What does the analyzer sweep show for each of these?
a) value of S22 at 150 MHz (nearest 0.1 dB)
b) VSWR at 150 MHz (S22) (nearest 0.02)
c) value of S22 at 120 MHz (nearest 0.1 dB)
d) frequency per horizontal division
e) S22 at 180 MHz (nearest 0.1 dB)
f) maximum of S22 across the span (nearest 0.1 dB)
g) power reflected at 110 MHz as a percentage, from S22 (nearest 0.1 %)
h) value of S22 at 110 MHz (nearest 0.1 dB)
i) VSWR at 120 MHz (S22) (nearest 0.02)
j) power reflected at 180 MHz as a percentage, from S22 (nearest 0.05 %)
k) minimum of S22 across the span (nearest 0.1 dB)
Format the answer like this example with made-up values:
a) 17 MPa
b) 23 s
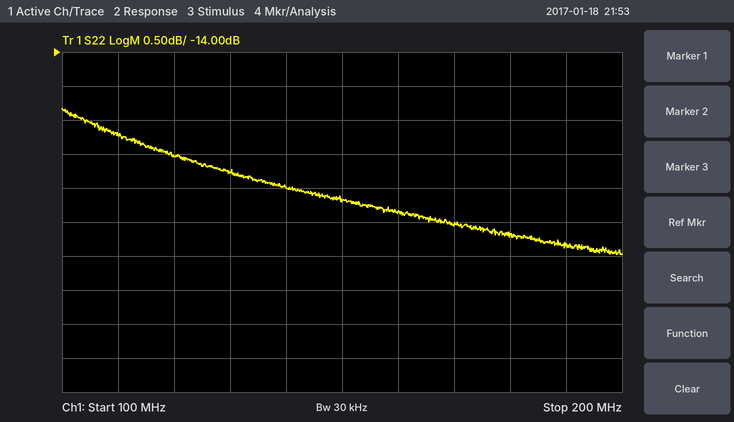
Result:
a) -16.2 dB
b) 1.36
c) -15.5 dB
d) 10 MHz
e) -16.7 dB
f) -14.8 dB
g) 3.0 %
h) -15.2 dB
i) 1.40
j) 2.15 %
k) -17.0 dB
